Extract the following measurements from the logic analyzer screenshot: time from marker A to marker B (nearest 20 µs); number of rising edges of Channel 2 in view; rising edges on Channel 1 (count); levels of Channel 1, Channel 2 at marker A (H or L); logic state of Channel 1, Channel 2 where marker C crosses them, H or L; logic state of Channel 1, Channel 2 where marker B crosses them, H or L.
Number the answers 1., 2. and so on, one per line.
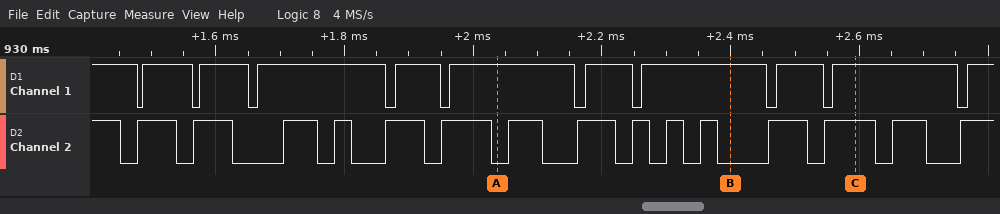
1. 360 µs
2. 15
3. 10
4. Channel 1=H, Channel 2=L
5. Channel 1=H, Channel 2=H
6. Channel 1=H, Channel 2=L
